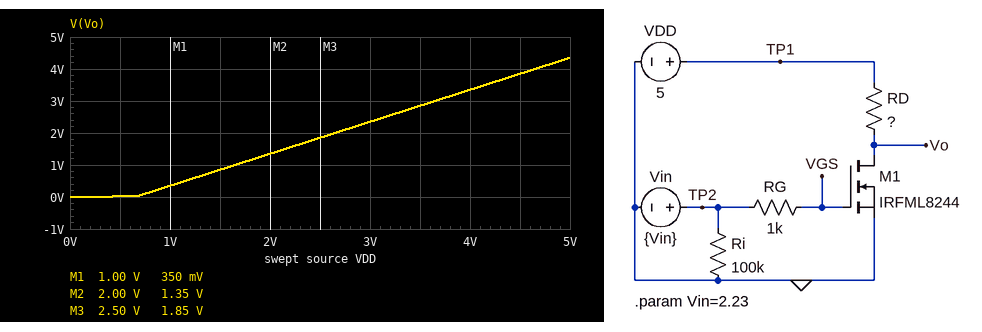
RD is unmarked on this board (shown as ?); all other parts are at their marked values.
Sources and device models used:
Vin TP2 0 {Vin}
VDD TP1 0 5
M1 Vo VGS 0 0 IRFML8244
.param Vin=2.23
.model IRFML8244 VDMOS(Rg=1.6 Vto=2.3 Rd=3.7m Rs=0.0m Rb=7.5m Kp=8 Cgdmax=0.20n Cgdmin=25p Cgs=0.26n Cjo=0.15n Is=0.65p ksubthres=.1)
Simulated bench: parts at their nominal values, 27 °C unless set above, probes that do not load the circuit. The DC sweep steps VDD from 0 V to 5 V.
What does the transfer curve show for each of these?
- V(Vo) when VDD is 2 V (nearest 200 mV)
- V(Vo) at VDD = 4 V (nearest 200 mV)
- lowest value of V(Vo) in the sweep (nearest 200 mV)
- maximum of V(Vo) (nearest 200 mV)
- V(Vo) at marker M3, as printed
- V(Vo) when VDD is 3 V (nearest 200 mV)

1.4 V
3.4 V
0 V
4.4 V
1.85 V
2.4 V
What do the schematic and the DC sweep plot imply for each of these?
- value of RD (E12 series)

100 Ω
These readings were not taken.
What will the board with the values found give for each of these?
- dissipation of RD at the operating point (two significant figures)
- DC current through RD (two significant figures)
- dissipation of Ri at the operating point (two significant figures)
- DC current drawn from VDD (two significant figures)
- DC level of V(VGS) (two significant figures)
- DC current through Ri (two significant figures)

4.2 mW
6.5 mA
50 µW
6.5 mA
2.2 V
22 µA
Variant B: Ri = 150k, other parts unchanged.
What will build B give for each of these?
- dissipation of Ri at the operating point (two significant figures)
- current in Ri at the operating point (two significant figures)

33 µW
15 µA
